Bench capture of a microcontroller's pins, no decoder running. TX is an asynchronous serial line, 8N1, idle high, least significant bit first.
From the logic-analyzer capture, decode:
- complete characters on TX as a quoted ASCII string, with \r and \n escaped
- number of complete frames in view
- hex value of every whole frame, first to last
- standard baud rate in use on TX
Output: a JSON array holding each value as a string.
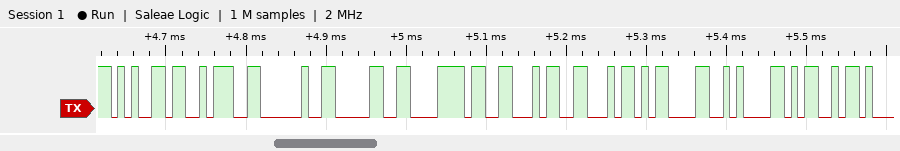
["\"e: 0xFF\\r\\nM\"", "10", "65 3A 20 30 78 46 46 0D 0A 4D", "115200 baud"]
